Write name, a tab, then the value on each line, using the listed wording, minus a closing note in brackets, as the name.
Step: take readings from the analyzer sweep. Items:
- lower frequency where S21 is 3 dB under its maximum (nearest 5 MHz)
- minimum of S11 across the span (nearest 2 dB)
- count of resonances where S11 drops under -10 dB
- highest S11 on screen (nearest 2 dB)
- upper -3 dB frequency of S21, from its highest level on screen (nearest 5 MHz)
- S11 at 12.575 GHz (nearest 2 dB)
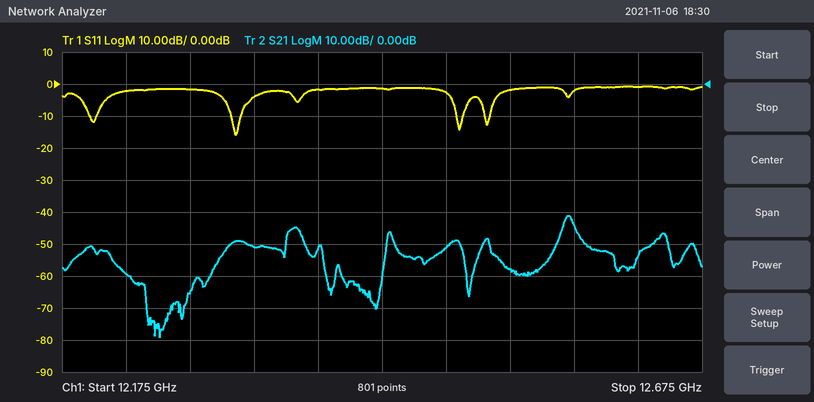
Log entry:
lower frequency where S21 is 3 dB under its maximum	12.565 GHz
minimum of S11 across the span	-16 dB
count of resonances where S11 drops under -10 dB	4
highest S11 on screen	0 dB
upper -3 dB frequency of S21, from its highest level on screen	12.575 GHz
S11 at 12.575 GHz	-2 dB
